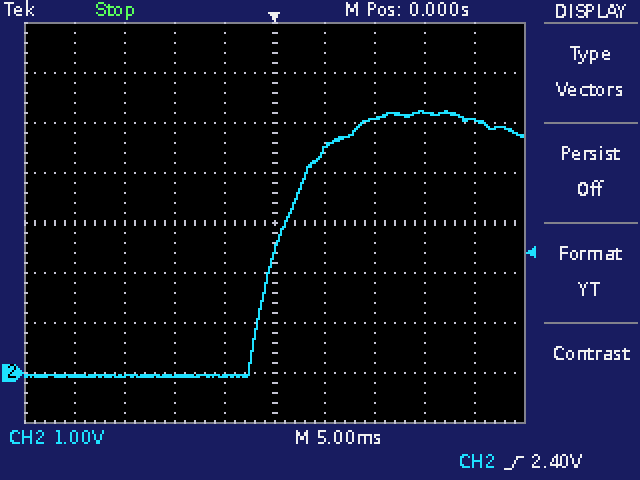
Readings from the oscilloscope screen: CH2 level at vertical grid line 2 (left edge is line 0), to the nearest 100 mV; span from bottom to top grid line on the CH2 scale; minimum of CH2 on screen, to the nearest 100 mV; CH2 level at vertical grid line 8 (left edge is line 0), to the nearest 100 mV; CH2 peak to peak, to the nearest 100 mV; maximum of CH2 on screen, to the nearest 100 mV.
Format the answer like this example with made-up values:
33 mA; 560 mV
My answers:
-100 mV; 8 V; -100 mV; 5.2 V; 5.3 V; 5.2 V
